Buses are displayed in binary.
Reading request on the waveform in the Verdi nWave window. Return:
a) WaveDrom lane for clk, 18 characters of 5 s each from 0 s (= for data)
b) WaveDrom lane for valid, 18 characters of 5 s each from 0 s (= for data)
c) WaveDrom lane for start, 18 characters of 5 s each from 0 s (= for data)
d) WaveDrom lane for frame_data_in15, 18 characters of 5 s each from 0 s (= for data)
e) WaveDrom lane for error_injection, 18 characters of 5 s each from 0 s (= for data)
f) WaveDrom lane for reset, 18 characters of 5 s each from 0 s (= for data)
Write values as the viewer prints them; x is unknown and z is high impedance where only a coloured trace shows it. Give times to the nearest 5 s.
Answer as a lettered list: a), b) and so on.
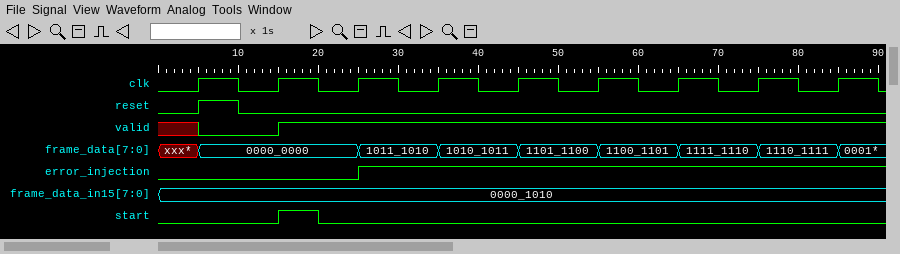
a) {name: 'clk', wave: '010101010101010101'}
b) {name: 'valid', wave: 'x0.1..............'}
c) {name: 'start', wave: '0..10.............'}
d) {name: 'frame_data_in15', wave: '=.................', data: '0000_1010'}
e) {name: 'error_injection', wave: '0....1............'}
f) {name: 'reset', wave: '010...............'}
